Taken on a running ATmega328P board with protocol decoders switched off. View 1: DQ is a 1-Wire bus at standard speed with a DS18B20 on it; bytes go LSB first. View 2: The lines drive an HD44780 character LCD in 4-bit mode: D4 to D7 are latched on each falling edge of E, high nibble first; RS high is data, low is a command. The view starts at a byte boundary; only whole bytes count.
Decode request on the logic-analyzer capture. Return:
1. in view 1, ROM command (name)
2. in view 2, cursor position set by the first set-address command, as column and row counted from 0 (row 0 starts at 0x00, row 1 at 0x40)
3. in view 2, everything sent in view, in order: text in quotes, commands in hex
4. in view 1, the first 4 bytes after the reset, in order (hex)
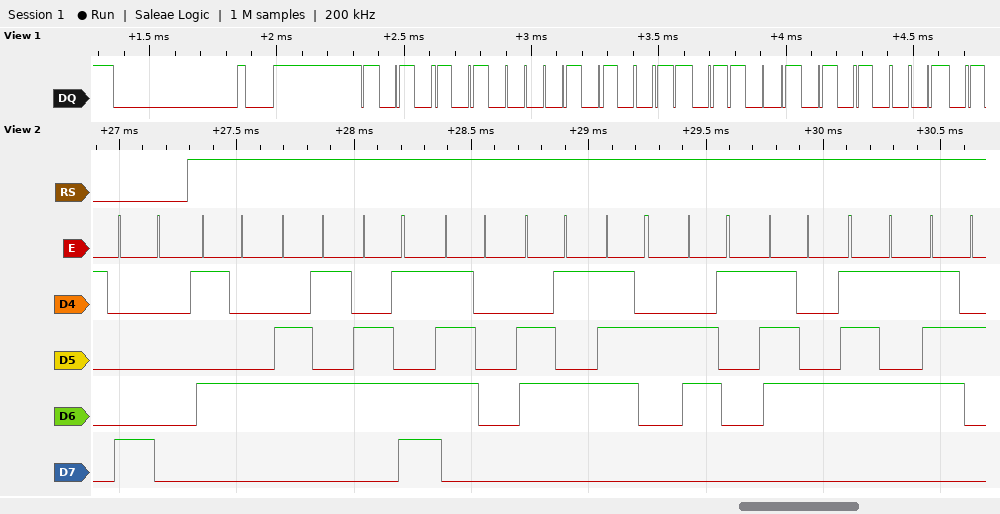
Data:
Match ROM
column 0, row 0
0x80 "Temperatur"
55 28 9B 8A
